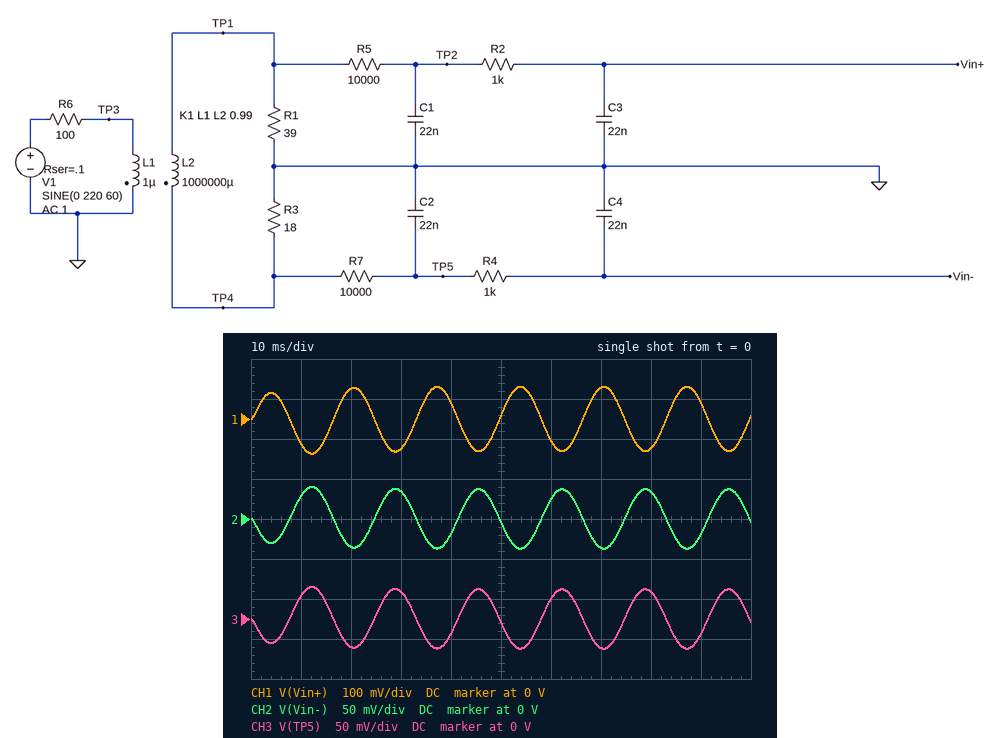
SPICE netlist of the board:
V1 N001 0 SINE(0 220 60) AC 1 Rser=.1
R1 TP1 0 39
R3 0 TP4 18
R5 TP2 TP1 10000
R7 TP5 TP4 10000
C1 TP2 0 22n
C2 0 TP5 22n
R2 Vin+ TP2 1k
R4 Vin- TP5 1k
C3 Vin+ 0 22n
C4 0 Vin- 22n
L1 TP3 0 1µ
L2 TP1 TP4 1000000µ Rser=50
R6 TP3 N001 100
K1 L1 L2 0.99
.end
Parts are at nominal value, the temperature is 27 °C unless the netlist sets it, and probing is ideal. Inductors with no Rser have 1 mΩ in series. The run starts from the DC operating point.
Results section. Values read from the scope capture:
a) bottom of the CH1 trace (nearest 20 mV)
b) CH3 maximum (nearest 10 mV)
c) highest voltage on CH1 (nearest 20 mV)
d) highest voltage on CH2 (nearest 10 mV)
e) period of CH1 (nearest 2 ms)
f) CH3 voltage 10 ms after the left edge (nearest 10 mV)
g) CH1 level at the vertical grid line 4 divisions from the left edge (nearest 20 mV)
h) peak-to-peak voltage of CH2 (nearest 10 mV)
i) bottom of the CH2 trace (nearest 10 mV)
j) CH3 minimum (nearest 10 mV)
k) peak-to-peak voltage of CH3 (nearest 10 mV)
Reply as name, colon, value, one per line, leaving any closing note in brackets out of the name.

bottom of the CH1 trace: -80 mV
CH3 maximum: 40 mV
highest voltage on CH1: 80 mV
highest voltage on CH2: 40 mV
period of CH1: 16 ms
CH3 voltage 10 ms after the left edge: 30 mV
CH1 level at the vertical grid line 4 divisions from the left edge: 40 mV
peak-to-peak voltage of CH2: 80 mV
bottom of the CH2 trace: -40 mV
CH3 minimum: -40 mV
peak-to-peak voltage of CH3: 80 mV
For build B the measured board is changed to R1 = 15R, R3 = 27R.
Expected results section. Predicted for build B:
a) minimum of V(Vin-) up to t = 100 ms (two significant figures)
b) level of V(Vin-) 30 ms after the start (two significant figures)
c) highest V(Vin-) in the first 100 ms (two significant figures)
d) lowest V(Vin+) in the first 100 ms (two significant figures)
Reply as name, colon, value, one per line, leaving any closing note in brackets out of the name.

minimum of V(Vin-) up to t = 100 ms: -56 mV
level of V(Vin-) 30 ms after the start: 53 mV
highest V(Vin-) in the first 100 ms: 61 mV
lowest V(Vin+) in the first 100 ms: -34 mV
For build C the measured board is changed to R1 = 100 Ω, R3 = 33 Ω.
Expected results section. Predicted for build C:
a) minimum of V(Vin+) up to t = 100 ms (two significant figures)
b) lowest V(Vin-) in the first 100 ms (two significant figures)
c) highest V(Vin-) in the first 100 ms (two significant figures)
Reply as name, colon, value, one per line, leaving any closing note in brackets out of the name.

minimum of V(Vin+) up to t = 100 ms: -200 mV
lowest V(Vin-) in the first 100 ms: -64 mV
highest V(Vin-) in the first 100 ms: 67 mV
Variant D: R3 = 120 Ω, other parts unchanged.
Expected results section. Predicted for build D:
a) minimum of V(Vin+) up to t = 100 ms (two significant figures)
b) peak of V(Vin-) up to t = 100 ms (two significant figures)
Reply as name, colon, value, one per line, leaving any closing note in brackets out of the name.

minimum of V(Vin+) up to t = 100 ms: -77 mV
peak of V(Vin-) up to t = 100 ms: 240 mV
